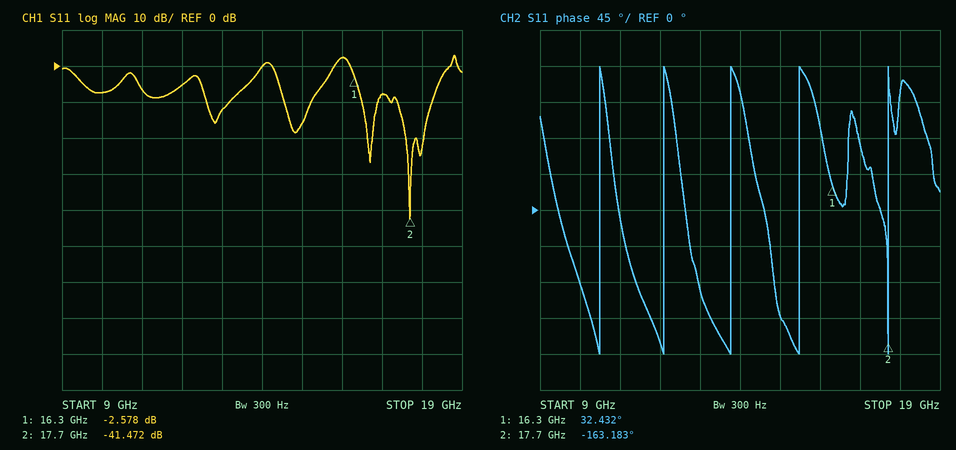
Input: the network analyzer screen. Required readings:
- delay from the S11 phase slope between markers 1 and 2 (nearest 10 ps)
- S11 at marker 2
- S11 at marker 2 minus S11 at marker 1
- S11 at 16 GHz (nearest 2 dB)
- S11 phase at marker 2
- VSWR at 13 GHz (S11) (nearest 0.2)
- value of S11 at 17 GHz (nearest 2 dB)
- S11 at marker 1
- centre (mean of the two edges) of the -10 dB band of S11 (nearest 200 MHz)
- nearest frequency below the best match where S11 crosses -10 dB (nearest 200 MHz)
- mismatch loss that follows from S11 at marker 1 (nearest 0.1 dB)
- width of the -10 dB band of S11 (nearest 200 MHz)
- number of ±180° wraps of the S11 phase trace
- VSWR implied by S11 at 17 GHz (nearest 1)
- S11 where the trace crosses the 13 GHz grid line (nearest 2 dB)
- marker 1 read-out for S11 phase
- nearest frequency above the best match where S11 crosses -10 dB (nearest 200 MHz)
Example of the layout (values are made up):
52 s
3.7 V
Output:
390 ps
-41.472 dB
-38.894 dB
2 dB
-163.183°
1.6
-8 dB
-2.578 dB
17.8 GHz
17.4 GHz
3.5 dB
800 MHz
5
2
-12 dB
32.432°
18.2 GHz
